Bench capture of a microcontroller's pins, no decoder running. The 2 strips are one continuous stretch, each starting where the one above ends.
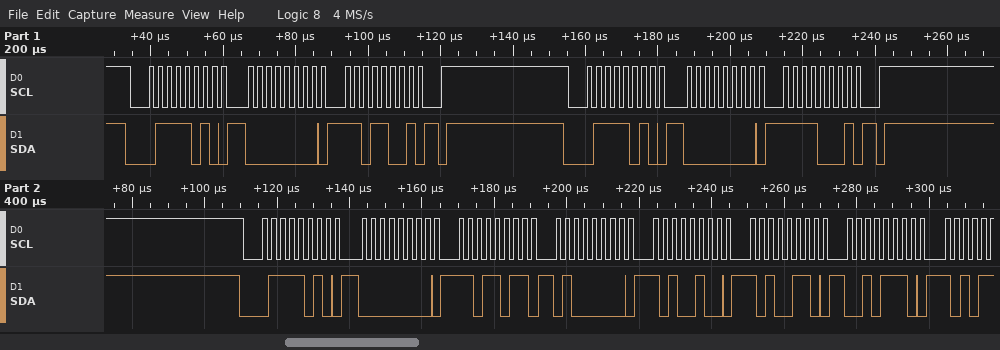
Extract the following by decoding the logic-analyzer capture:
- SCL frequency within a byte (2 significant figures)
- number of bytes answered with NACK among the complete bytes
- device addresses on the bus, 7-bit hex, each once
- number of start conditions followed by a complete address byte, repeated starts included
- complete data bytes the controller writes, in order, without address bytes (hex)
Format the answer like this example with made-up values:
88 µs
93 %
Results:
400 kHz
0
0x3D
3
00 D9 00 F1 00 DB 40 A4 A6 2E
